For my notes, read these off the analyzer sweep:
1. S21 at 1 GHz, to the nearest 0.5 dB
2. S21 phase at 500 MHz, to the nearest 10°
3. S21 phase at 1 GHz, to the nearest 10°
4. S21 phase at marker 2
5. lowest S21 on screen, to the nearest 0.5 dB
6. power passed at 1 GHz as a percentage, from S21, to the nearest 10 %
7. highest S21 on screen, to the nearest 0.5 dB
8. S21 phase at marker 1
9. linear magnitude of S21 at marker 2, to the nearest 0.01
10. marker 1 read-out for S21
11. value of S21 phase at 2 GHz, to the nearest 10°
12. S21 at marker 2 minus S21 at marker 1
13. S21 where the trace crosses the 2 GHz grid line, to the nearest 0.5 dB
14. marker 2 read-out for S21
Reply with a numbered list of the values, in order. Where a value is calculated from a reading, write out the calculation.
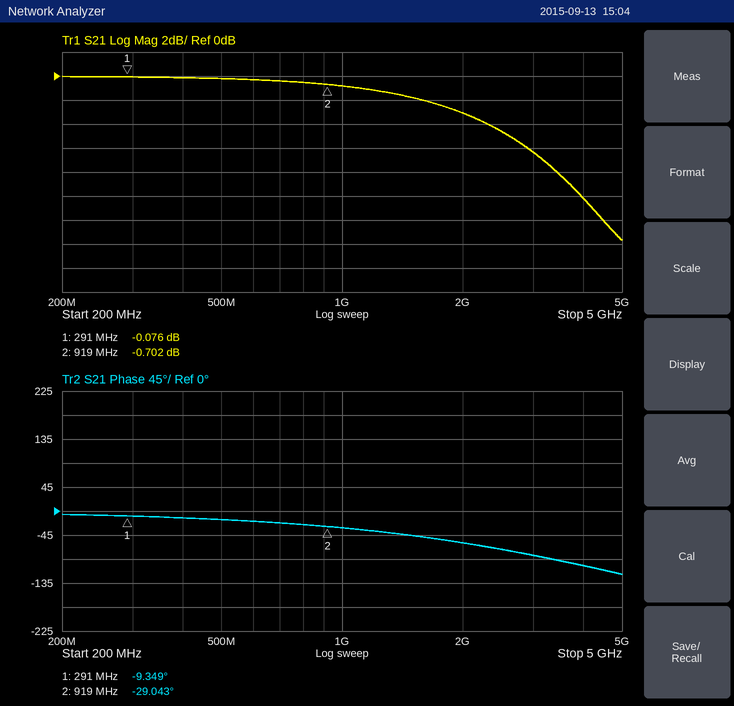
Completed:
1. -1.0 dB
2. -20°
3. -30°
4. -29.043°
5. -13.5 dB
6. 10^(-1/10) ≈ 79.4 %, so 80 % to the nearest 10 %
7. 0.0 dB
8. -9.349°
9. 10^(-0.702/20) ≈ 0.92
10. -0.076 dB
11. -60°
12. -0.702 − (-0.076) = -0.626 dB
13. -3.0 dB
14. -0.702 dB
